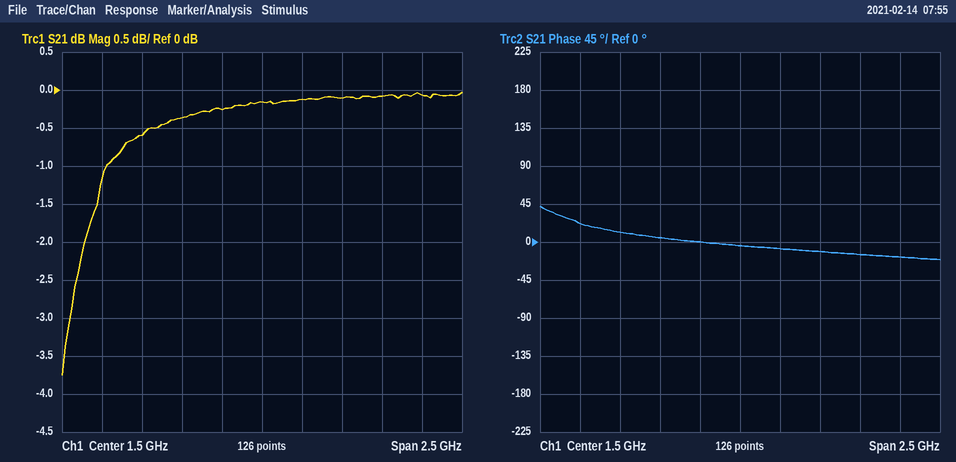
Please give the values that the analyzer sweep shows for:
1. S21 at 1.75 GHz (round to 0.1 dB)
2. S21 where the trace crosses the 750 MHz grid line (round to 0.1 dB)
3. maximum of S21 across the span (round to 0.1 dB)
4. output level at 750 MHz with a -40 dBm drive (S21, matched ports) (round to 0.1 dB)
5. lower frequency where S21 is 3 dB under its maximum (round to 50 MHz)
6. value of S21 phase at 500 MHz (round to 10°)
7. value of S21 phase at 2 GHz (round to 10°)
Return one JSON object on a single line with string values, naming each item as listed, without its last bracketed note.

{"S21 at 1.75 GHz": "-0.1 dB", "S21 where the trace crosses the 750 MHz grid line": "-0.6 dB", "maximum of S21 across the span": "0.0 dB", "output level at 750 MHz with a -40 dBm drive (S21, matched ports)": "-40.6 dBm", "lower frequency where S21 is 3 dB under its maximum": "300 MHz", "value of S21 phase at 500 MHz": "20°", "value of S21 phase at 2 GHz": "-10°"}
